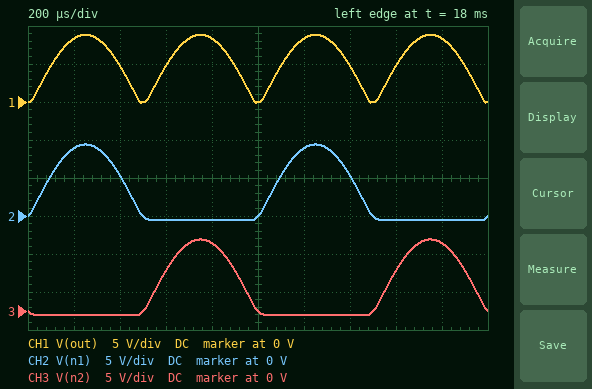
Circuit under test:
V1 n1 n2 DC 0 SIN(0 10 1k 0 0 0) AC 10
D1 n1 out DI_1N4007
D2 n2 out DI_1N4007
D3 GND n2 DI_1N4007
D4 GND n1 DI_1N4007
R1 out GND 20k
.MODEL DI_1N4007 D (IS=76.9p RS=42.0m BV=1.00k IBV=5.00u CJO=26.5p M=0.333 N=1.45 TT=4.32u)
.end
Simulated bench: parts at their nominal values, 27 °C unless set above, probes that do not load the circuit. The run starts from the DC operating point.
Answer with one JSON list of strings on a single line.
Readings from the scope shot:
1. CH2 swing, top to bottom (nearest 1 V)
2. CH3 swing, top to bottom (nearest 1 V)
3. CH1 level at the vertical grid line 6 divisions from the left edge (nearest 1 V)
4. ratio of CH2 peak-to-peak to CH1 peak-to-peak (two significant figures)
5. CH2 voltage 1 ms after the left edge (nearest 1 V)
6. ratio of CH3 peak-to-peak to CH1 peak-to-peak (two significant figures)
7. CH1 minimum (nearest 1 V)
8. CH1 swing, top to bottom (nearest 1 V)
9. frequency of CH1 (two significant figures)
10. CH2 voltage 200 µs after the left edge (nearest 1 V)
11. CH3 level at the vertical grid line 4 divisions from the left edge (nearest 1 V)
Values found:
["10 V", "10 V", "8 V", "1.1", "0 V", "1.1", "0 V", "9 V", "2.0 kHz", "9 V", "9 V"]
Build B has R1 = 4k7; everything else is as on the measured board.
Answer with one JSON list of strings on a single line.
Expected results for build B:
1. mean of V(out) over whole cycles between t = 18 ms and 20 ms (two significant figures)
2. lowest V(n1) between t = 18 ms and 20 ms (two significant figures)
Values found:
["5.2 V", "-640 mV"]
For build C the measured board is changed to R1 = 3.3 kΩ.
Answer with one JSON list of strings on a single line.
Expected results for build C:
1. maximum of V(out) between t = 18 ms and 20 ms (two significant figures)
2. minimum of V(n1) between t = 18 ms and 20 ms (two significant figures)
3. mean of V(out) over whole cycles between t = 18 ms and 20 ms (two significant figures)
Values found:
["8.7 V", "-650 mV", "5.2 V"]
